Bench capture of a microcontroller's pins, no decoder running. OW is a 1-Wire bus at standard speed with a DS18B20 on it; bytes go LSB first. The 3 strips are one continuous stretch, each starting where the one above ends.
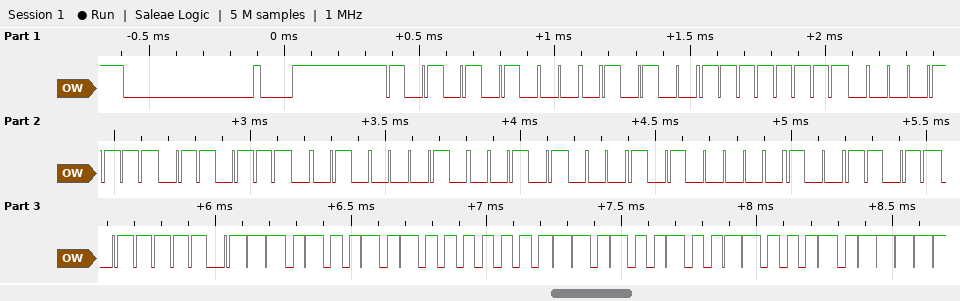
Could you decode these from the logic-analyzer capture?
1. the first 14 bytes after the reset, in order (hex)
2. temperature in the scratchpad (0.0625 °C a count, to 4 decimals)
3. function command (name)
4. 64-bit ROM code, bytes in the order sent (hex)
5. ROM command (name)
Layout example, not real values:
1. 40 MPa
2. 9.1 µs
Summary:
1. 55 28 FF F0 76 42 14 05 D9 BE 4B 01 4B 46
2. 20.6875 °C
3. Read Scratchpad
4. 28 FF F0 76 42 14 05 D9
5. Match ROM
